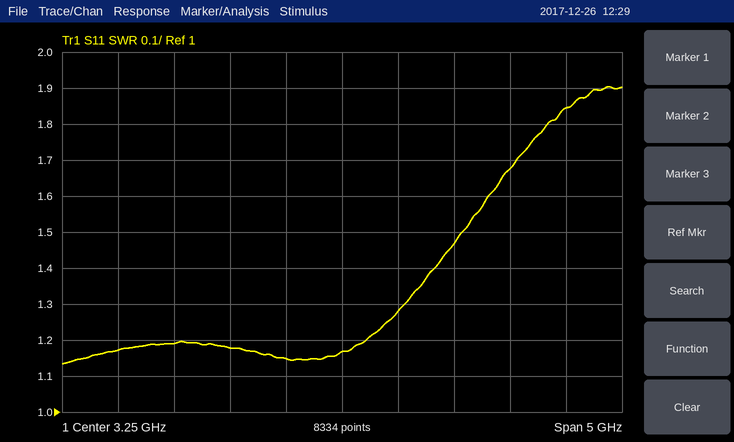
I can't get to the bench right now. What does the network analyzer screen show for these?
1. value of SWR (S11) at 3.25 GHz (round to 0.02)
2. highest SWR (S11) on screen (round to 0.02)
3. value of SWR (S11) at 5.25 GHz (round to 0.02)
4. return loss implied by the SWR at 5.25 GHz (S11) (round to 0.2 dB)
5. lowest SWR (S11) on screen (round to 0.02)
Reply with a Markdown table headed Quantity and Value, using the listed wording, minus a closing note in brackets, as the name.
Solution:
| Quantity | Value |
|---|---|
| value of SWR (S11) at 3.25 GHz | 1.16 |
| highest SWR (S11) on screen | 1.90 |
| value of SWR (S11) at 5.25 GHz | 1.84 |
| return loss implied by the SWR at 5.25 GHz (S11) | 10.6 dB |
| lowest SWR (S11) on screen | 1.14 |
